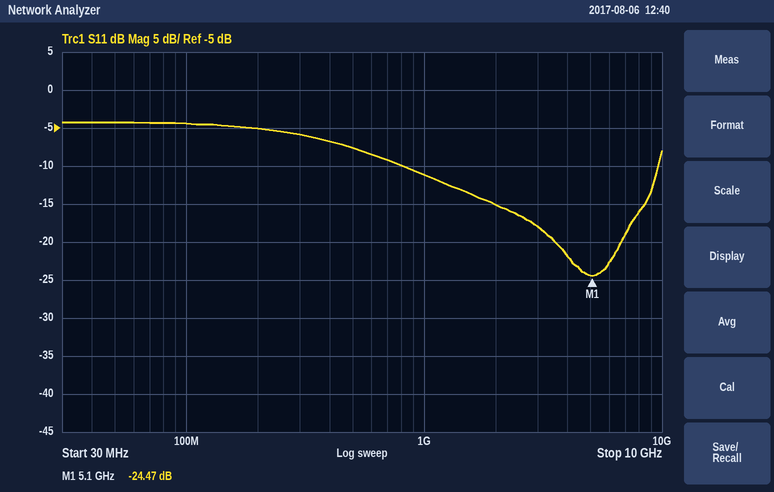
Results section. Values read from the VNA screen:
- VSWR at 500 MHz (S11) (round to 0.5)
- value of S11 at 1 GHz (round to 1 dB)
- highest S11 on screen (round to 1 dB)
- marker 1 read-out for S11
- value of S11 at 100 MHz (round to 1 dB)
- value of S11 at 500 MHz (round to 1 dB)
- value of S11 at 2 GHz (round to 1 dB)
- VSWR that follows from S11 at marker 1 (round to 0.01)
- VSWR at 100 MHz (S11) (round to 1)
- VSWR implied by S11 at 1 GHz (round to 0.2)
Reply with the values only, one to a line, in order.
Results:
2.5
-11 dB
-4 dB
-24.47 dB
-4 dB
-8 dB
-15 dB
1.13
4
1.8
